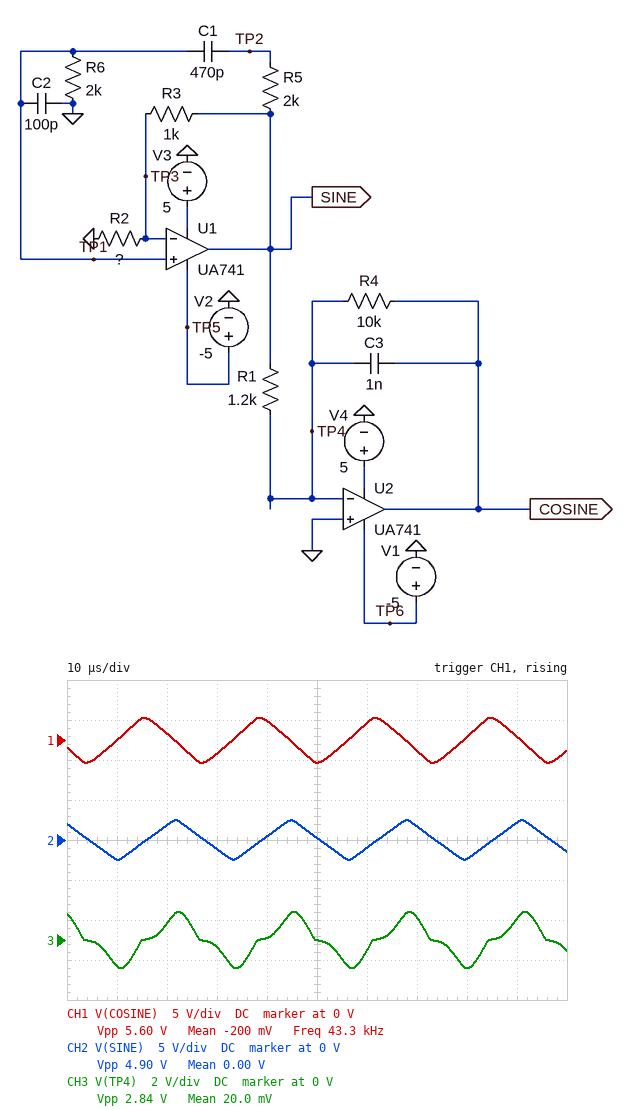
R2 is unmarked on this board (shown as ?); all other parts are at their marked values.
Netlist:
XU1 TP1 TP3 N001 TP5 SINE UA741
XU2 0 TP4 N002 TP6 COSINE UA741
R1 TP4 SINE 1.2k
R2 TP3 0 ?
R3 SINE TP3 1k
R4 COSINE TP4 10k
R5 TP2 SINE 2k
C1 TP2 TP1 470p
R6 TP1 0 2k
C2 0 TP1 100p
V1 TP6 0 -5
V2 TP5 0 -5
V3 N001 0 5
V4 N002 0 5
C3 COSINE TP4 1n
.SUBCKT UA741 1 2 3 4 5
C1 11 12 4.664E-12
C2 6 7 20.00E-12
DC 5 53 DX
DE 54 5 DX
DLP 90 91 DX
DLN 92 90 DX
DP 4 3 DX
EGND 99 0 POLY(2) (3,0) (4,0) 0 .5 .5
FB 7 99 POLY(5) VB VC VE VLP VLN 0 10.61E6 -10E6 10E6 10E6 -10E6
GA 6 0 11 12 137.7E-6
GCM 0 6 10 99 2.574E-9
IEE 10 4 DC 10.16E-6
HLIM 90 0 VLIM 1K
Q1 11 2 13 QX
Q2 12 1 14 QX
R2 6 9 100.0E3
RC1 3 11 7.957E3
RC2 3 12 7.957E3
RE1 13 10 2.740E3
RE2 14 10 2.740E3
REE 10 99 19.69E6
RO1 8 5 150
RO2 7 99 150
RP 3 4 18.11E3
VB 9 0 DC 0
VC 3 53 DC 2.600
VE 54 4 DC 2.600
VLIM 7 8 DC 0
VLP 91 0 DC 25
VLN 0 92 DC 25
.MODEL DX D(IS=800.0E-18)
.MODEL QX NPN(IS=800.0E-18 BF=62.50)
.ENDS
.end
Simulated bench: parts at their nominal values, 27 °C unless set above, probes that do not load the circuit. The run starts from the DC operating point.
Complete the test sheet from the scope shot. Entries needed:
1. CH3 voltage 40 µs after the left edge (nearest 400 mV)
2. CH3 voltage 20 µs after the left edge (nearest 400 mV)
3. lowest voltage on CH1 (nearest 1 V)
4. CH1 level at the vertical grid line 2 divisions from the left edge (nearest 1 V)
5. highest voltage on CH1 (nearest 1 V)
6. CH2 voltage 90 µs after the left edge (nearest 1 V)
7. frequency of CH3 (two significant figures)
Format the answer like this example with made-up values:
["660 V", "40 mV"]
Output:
["0 V", "800 mV", "-3 V", "1 V", "3 V", "2 V", "43 kHz"]
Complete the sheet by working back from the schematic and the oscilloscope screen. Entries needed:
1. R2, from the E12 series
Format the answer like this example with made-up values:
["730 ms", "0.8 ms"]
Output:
["180 Ω"]
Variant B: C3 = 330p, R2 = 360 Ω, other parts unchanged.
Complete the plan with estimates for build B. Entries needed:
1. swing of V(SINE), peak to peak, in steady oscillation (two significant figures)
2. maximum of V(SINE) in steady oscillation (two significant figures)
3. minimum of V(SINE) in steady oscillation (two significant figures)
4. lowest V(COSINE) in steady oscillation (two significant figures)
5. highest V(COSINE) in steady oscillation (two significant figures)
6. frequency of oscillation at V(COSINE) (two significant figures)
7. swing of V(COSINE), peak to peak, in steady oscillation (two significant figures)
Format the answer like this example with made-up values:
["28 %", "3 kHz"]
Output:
["2.7 V", "1.3 V", "-1.3 V", "-1.6 V", "1.6 V", "77 kHz", "3.2 V"]
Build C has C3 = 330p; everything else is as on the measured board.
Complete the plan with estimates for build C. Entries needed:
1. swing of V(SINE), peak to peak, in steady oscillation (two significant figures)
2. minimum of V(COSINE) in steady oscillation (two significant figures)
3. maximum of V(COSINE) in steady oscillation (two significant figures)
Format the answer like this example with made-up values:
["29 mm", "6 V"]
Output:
["5.0 V", "-3.0 V", "2.7 V"]
